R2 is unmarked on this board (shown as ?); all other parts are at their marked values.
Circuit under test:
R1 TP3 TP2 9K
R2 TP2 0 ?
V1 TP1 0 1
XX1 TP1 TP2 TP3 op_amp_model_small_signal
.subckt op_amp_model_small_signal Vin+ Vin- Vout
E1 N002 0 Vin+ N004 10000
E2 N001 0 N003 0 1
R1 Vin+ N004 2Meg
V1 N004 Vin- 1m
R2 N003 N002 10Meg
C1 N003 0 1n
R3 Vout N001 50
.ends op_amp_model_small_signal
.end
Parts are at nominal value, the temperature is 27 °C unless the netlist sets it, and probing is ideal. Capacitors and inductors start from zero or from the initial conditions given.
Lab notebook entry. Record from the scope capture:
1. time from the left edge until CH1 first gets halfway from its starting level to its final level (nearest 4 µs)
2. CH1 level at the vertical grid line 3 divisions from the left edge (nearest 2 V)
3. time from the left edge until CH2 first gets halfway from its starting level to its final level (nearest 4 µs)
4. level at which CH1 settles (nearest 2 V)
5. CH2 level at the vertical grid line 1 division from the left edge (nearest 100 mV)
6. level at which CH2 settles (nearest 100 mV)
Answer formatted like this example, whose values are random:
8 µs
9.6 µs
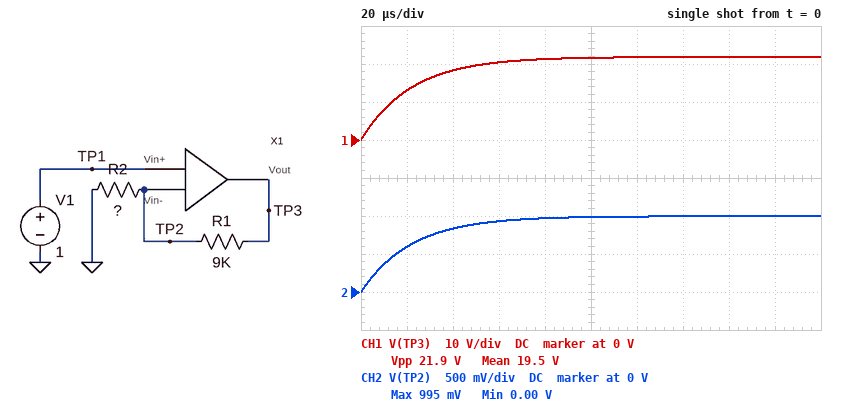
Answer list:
16 µs
20 V
16 µs
22 V
600 mV
1.0 V
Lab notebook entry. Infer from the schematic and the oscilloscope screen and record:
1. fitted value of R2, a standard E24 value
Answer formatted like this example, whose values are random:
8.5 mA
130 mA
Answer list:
430 Ω
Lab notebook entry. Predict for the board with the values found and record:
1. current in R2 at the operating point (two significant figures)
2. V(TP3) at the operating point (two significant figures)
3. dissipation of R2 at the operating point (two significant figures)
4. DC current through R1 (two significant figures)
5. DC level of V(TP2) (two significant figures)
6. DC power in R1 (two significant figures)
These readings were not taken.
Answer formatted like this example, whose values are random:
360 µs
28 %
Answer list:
2.3 mA
22 V
2.3 mW
2.3 mA
1.0 V
48 mW
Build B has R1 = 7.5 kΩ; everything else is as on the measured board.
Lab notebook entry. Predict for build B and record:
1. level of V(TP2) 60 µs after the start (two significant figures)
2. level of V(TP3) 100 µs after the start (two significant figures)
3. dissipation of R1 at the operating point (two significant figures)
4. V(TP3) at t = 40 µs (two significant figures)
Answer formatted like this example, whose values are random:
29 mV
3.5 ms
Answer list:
960 mV
18 V
40 mW
16 V
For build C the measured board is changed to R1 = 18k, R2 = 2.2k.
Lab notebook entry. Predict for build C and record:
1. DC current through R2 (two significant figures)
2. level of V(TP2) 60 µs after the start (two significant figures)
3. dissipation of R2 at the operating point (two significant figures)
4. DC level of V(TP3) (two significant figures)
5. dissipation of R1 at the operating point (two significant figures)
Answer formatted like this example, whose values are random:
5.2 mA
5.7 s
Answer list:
450 µA
1.0 V
450 µW
9.2 V
3.7 mW
